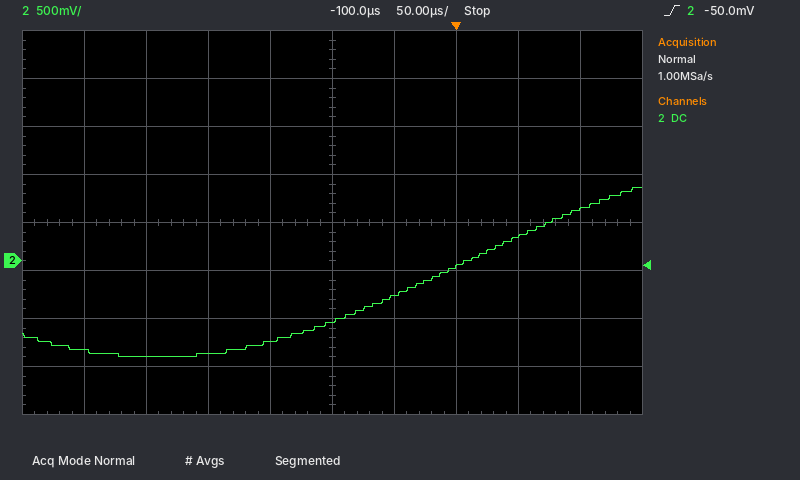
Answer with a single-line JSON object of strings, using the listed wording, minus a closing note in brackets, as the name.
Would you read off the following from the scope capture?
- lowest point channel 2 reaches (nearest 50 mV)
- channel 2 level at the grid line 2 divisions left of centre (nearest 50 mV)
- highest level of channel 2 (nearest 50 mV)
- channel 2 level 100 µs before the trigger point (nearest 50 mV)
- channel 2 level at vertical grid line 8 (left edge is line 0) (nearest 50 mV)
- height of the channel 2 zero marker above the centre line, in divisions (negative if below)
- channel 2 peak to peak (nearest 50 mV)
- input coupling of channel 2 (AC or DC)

{"lowest point channel 2 reaches": "-1.00 V", "channel 2 level at the grid line 2 divisions left of centre": "-950 mV", "highest level of channel 2": "750 mV", "channel 2 level 100 µs before the trigger point": "-650 mV", "channel 2 level at vertical grid line 8 (left edge is line 0)": "250 mV", "height of the channel 2 zero marker above the centre line, in divisions": "-0.8 div", "channel 2 peak to peak": "1.75 V", "input coupling of channel 2": "DC"}
